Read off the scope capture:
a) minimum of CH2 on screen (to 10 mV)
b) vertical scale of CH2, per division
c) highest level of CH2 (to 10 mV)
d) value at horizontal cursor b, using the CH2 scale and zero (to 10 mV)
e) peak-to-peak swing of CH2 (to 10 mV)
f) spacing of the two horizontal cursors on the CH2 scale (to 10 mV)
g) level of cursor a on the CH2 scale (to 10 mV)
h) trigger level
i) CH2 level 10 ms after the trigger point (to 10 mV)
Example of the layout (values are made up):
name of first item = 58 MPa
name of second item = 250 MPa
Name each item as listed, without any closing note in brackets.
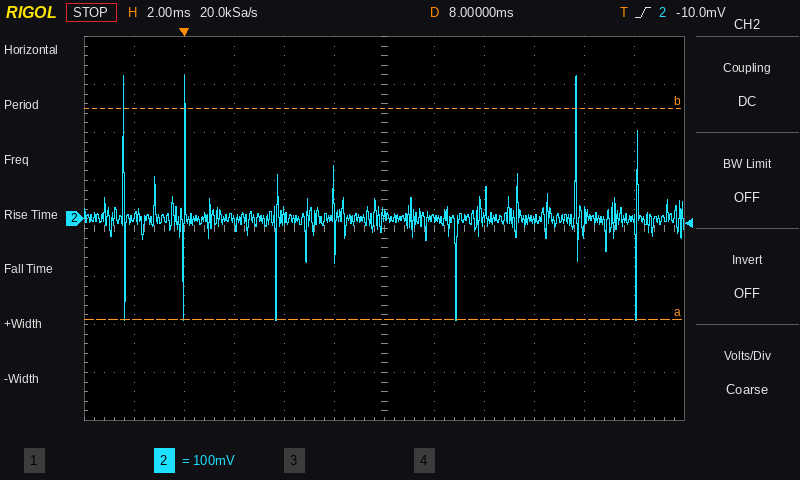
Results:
minimum of CH2 on screen = -210 mV
vertical scale of CH2, per division = 100 mV
highest level of CH2 = 300 mV
value at horizontal cursor b, using the CH2 scale and zero = 230 mV
peak-to-peak swing of CH2 = 510 mV
spacing of the two horizontal cursors on the CH2 scale = 440 mV
level of cursor a on the CH2 scale = -210 mV
trigger level = -10.0 mV
CH2 level 10 ms after the trigger point = 0 mV
